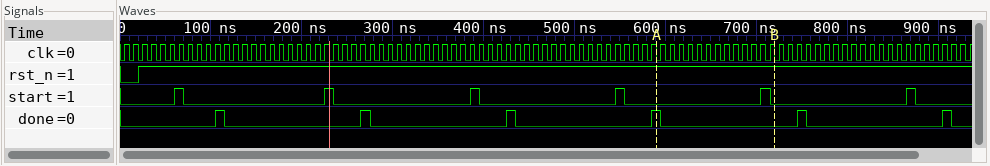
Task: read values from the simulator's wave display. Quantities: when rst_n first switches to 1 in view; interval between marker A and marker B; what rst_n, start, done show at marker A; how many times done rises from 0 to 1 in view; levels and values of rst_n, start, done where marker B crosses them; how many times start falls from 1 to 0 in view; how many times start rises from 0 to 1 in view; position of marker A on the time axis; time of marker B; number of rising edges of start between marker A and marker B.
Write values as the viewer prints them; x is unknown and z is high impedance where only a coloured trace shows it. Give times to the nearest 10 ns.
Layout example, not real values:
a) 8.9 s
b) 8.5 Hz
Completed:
a) 20 ns
b) 130 ns
c) rst_n=1, start=0, done=1
d) 6
e) rst_n=1, start=0, done=0
f) 6
g) 6
h) 590 ns
i) 720 ns
j) 1
